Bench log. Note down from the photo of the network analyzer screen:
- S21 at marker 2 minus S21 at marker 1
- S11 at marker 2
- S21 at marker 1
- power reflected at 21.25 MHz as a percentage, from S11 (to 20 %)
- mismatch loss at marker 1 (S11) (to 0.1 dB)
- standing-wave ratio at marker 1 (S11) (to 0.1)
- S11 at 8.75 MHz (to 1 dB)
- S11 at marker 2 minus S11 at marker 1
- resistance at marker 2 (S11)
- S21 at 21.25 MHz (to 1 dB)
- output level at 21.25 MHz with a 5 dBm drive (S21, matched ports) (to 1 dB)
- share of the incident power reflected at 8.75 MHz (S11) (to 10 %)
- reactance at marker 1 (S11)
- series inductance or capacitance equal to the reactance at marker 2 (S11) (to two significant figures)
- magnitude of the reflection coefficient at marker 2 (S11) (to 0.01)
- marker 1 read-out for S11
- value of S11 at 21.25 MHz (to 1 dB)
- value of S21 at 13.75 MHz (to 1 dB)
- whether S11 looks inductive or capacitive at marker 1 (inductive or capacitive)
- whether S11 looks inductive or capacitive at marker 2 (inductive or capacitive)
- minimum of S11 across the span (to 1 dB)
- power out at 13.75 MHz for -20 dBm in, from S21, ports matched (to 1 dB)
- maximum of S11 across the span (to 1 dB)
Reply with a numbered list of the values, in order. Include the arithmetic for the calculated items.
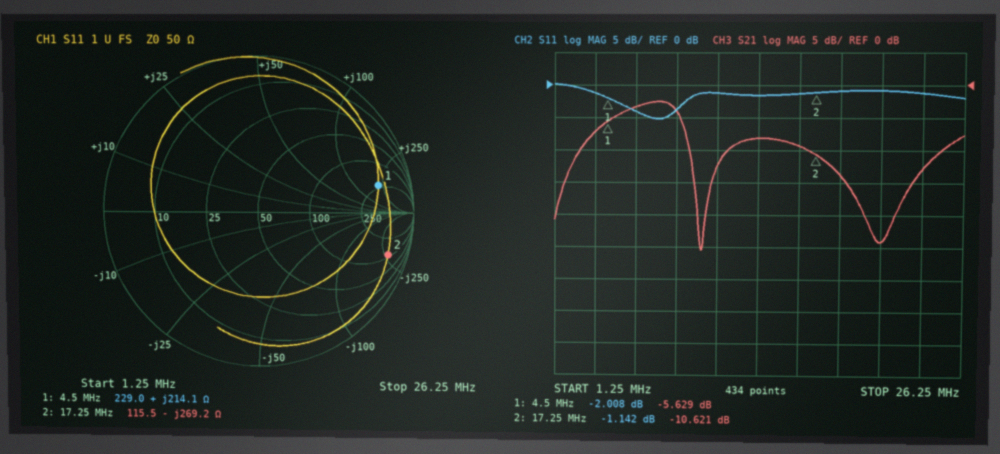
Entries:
1. -10.621 − (-5.629) = -4.992 dB
2. -1.142 dB
3. -5.629 dB
4. 10^(-1/10) ≈ 79.4 %, so 80 % to the nearest 20 %
5. −10 log10(1 − 10^(-2.008/10)) ≈ 4.3 dB
6. 8.7
7. -4 dB
8. -1.142 − (-2.008) = 0.866 dB
9. 115.5 Ω
10. -24 dB
11. 5 dBm + (-24 dB) = -19 dBm
12. 10^(-4/10) ≈ 40 %
13. +214.1 Ω
14. C = 1/(2π × 17.25 MHz × 269.2 Ω) ≈ 34 pF
15. 0.88
16. -2.008 dB
17. -1 dB
18. -8 dB
19. inductive
20. capacitive
21. -5 dB
22. -20 dBm + (-8 dB) = -28 dBm
23. 0 dB
